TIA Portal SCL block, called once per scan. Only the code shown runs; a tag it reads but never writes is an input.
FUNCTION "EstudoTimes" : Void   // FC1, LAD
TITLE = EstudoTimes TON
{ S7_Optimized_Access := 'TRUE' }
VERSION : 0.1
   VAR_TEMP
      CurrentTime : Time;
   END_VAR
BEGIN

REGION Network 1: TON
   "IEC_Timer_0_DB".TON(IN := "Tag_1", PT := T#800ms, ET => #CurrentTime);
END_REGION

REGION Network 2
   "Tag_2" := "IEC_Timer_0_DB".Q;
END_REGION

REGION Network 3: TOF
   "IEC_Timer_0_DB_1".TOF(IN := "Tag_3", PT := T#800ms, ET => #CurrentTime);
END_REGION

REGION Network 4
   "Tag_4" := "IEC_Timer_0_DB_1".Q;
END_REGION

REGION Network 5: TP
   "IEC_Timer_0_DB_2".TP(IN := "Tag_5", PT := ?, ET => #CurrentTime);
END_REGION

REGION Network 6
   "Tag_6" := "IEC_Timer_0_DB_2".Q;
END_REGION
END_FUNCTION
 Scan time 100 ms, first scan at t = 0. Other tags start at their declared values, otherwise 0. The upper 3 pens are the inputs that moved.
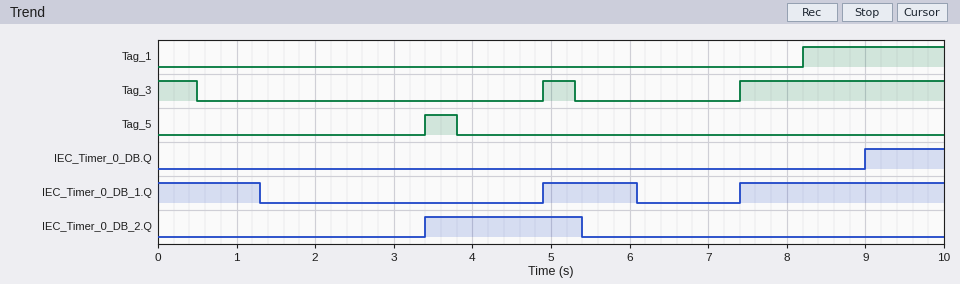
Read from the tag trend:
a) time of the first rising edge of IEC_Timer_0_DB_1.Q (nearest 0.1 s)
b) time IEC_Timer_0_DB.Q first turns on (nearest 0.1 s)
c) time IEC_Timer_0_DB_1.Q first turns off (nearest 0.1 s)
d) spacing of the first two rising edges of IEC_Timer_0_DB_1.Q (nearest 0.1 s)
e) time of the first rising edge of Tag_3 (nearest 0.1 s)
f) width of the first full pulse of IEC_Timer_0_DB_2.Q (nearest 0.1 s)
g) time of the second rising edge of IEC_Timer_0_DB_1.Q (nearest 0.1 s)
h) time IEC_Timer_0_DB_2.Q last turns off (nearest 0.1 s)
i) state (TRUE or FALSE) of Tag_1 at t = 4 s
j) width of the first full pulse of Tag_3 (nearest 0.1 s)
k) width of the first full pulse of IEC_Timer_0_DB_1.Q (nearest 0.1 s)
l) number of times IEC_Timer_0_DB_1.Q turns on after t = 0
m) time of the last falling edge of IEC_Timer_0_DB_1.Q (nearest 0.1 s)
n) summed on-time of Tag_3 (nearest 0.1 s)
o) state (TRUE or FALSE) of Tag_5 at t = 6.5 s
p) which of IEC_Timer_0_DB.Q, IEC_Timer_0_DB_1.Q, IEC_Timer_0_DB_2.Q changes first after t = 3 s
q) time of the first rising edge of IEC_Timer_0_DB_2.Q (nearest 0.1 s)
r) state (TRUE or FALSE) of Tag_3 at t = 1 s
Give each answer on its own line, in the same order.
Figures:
4.9 s
9.0 s
1.3 s
2.5 s
4.9 s
2.0 s
7.4 s
5.4 s
FALSE
0.4 s
1.2 s
2
6.1 s
3.5 s
FALSE
IEC_Timer_0_DB_2.Q
3.4 s
FALSE
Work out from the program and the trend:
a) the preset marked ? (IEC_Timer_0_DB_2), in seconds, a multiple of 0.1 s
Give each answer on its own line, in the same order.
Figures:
2.0 s
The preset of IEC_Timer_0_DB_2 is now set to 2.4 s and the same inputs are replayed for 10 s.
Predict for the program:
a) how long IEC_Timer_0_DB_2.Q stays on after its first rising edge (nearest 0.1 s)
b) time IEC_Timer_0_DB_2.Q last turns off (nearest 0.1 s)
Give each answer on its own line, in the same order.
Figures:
2.4 s
5.8 s
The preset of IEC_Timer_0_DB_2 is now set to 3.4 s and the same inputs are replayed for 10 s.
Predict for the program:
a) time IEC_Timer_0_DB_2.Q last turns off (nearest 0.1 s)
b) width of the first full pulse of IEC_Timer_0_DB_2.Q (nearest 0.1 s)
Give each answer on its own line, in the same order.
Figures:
6.8 s
3.4 s
